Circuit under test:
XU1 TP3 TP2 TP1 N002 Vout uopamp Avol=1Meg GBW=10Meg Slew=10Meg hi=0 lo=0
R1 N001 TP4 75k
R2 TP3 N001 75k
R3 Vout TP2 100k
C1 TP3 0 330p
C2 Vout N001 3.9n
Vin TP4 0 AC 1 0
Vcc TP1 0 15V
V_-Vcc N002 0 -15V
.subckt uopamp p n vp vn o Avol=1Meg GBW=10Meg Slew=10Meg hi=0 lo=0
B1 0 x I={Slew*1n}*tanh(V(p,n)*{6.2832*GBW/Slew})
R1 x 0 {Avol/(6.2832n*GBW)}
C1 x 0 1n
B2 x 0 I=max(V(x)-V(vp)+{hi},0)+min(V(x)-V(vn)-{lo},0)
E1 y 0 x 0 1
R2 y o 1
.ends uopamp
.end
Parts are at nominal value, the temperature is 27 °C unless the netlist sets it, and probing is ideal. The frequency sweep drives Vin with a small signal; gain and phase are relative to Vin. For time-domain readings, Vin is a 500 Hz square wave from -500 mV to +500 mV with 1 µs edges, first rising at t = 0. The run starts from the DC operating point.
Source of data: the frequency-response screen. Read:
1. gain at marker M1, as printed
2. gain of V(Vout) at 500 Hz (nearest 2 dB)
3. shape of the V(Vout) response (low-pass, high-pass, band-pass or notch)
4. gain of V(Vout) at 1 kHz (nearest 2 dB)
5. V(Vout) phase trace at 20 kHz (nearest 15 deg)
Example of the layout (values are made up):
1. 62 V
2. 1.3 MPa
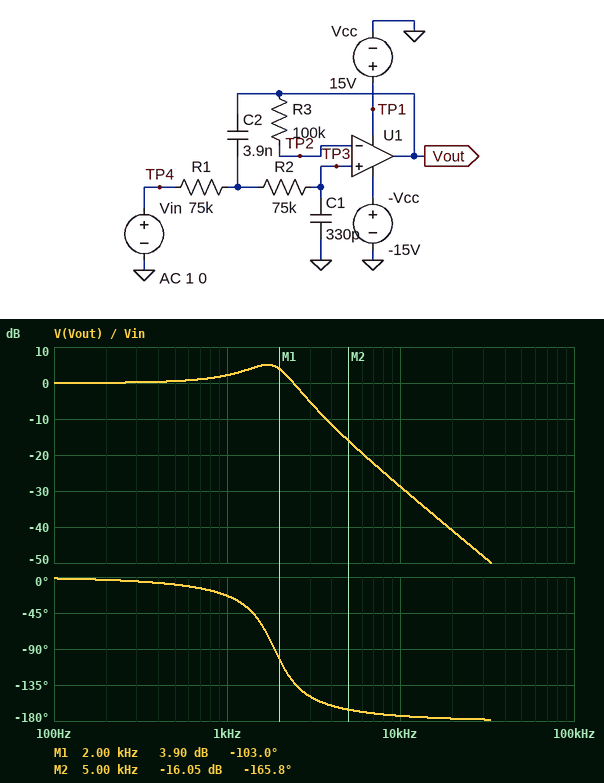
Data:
1. 3.90 dB
2. 0 dB
3. low-pass
4. 2 dB
5. -180 deg
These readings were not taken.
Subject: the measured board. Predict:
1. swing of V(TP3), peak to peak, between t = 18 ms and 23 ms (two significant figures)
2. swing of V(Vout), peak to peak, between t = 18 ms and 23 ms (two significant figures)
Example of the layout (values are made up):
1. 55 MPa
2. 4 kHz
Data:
1. 1.8 V
2. 1.8 V
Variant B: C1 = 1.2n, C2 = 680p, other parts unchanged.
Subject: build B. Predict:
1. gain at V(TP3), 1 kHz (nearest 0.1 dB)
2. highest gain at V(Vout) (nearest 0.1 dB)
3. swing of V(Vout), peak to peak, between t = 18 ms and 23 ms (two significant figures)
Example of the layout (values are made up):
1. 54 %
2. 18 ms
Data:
1. -2.9 dB
2. 0 dB
3. 1.0 V
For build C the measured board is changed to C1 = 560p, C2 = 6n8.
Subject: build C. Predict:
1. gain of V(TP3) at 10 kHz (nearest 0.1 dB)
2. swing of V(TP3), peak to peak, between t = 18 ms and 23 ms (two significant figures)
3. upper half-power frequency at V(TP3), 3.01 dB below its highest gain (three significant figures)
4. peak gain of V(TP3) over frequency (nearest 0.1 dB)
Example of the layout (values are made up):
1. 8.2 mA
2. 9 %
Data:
1. -38.5 dB
2. 1.7 V
3. 1.28 kHz
4. 5.2 dB
